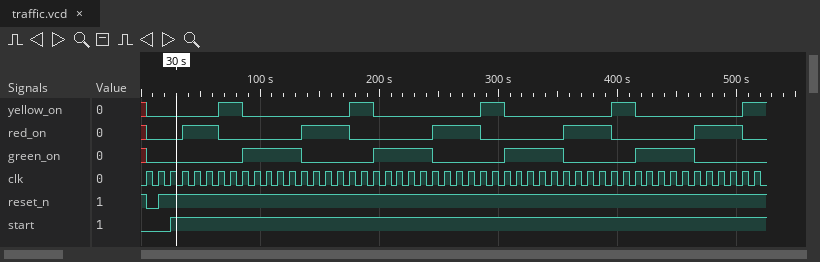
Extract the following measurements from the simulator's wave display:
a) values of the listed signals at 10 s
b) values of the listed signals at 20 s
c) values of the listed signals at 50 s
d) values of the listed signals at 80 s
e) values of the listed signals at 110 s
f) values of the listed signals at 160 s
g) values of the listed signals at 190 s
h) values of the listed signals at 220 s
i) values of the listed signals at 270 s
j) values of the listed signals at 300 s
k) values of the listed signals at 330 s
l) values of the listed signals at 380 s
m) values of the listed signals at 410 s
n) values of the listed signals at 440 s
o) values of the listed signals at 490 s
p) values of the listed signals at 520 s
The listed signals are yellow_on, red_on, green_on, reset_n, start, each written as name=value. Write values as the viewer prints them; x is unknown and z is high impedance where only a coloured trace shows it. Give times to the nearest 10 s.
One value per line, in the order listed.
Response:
yellow_on=0, red_on=0, green_on=0, reset_n=0, start=0
yellow_on=0, red_on=0, green_on=0, reset_n=1, start=0
yellow_on=0, red_on=1, green_on=0, reset_n=1, start=1
yellow_on=1, red_on=0, green_on=0, reset_n=1, start=1
yellow_on=0, red_on=0, green_on=1, reset_n=1, start=1
yellow_on=0, red_on=1, green_on=0, reset_n=1, start=1
yellow_on=1, red_on=0, green_on=0, reset_n=1, start=1
yellow_on=0, red_on=0, green_on=1, reset_n=1, start=1
yellow_on=0, red_on=1, green_on=0, reset_n=1, start=1
yellow_on=1, red_on=0, green_on=0, reset_n=1, start=1
yellow_on=0, red_on=0, green_on=1, reset_n=1, start=1
yellow_on=0, red_on=1, green_on=0, reset_n=1, start=1
yellow_on=1, red_on=0, green_on=0, reset_n=1, start=1
yellow_on=0, red_on=0, green_on=1, reset_n=1, start=1
yellow_on=0, red_on=1, green_on=0, reset_n=1, start=1
yellow_on=1, red_on=0, green_on=0, reset_n=1, start=1
